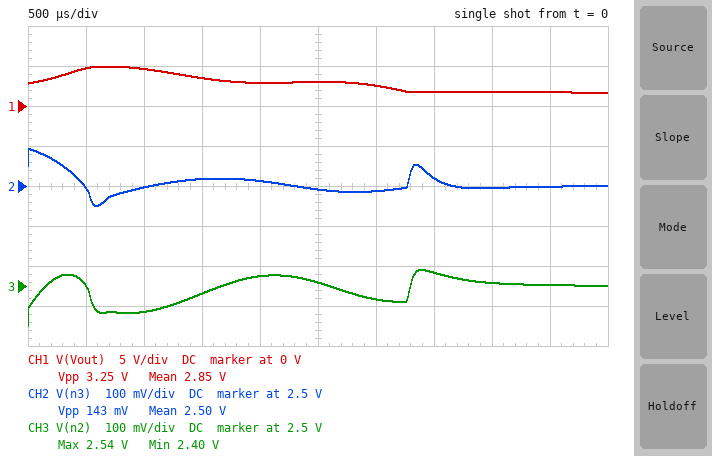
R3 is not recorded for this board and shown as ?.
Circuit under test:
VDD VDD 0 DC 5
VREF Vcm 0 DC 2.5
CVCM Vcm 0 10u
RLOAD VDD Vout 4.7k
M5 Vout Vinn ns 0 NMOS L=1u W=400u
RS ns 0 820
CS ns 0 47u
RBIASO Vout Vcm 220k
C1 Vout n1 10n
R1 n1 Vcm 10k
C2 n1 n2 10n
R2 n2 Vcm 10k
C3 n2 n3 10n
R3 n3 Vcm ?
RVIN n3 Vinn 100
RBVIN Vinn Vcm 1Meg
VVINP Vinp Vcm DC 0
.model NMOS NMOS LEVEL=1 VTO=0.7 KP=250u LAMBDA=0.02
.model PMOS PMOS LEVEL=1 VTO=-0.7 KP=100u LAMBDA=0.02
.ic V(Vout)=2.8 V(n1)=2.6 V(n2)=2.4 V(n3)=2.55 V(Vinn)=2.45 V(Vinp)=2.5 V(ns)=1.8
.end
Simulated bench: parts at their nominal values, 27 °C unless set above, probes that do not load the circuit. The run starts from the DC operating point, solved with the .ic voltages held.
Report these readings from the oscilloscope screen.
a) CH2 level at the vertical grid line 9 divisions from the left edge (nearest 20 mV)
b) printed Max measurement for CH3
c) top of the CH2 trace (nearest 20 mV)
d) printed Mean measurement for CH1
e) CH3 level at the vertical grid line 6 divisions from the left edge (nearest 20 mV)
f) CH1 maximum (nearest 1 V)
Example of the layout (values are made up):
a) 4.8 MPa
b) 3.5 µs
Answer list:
a) 2.50 V
b) 2.54 V
c) 2.60 V
d) 2.85 V
e) 2.46 V
f) 5 V
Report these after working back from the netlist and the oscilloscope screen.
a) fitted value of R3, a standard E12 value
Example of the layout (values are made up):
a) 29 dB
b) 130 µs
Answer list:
a) 18 kΩ
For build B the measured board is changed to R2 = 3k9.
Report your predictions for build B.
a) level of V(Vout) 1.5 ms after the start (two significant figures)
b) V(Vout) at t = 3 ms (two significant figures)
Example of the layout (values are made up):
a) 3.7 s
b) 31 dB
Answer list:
a) 3.8 V
b) 1.8 V
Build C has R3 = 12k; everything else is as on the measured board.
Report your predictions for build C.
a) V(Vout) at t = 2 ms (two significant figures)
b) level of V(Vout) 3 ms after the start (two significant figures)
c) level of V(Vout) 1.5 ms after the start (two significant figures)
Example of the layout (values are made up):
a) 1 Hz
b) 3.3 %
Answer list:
a) 3.4 V
b) 1.7 V
c) 3.6 V
